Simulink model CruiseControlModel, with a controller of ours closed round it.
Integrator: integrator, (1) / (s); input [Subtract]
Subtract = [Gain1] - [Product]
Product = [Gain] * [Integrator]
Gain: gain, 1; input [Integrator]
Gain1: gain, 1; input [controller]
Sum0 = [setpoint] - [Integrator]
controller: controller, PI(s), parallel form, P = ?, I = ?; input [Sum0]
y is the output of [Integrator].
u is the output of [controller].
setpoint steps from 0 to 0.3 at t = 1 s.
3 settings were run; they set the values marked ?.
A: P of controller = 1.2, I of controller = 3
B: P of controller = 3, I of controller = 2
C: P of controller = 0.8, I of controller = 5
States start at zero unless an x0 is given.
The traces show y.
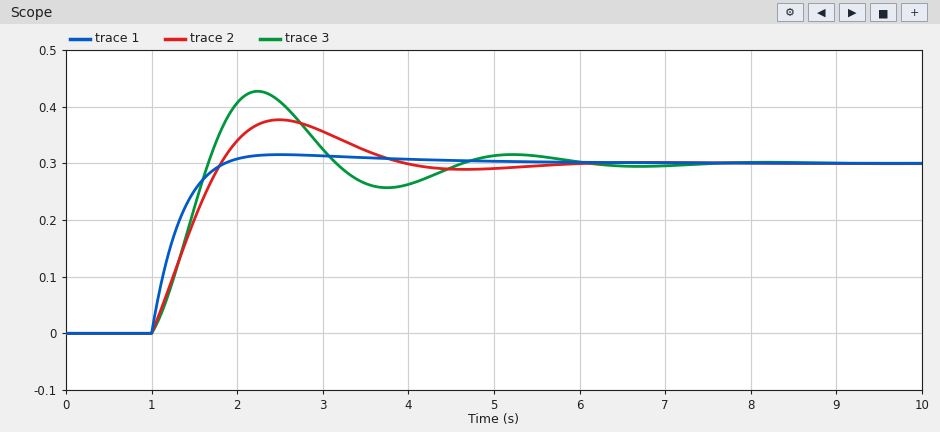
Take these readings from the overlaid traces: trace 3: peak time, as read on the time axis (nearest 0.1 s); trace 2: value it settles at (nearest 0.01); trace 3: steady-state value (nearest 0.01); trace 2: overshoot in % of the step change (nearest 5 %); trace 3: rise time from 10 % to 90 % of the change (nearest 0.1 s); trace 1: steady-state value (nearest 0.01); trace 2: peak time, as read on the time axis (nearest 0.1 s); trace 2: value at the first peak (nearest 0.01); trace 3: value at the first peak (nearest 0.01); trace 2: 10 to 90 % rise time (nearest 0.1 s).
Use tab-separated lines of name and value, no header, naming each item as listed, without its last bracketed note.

trace 3: peak time, as read on the time axis	2.2 s
trace 2: value it settles at	0.30
trace 3: steady-state value	0.30
trace 2: overshoot in % of the step change	25 %
trace 3: rise time from 10 % to 90 % of the change	0.5 s
trace 1: steady-state value	0.30
trace 2: peak time, as read on the time axis	2.5 s
trace 2: value at the first peak	0.38
trace 3: value at the first peak	0.43
trace 2: 10 to 90 % rise time	0.6 s
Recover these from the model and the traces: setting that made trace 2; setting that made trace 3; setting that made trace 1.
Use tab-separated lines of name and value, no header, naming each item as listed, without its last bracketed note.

setting that made trace 2	A
setting that made trace 3	C
setting that made trace 1	B
